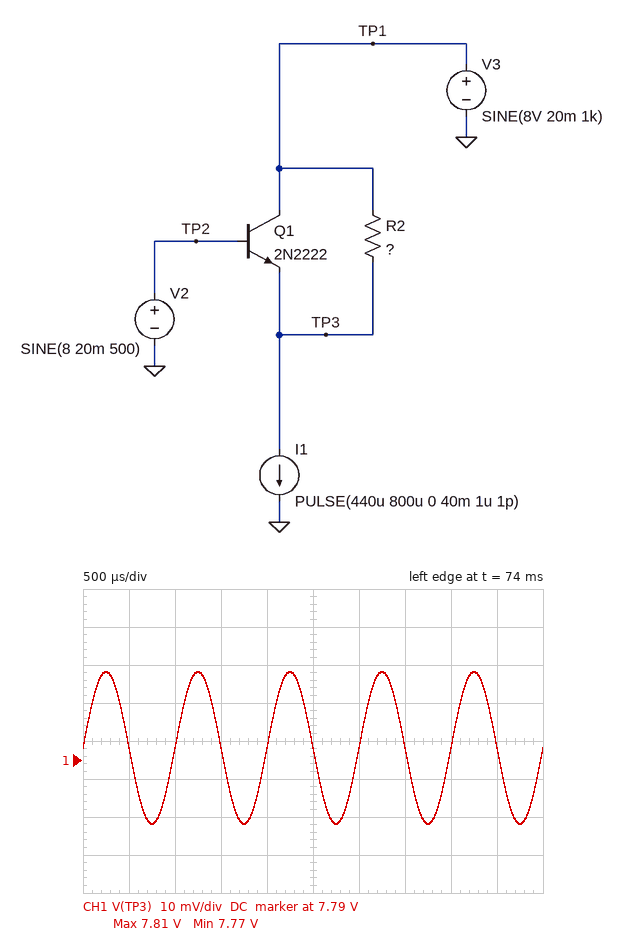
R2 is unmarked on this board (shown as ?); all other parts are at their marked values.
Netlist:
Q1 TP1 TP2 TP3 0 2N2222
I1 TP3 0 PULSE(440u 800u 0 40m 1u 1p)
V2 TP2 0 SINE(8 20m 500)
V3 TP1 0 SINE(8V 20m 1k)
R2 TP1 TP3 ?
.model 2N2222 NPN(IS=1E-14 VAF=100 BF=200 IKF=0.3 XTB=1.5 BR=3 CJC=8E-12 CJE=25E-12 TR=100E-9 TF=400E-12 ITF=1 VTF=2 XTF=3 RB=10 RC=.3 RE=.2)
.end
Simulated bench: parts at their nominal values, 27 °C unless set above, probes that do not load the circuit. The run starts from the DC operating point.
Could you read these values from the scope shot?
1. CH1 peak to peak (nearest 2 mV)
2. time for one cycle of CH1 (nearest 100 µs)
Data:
40 mV
1.0 ms
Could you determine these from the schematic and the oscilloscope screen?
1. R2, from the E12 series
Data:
470 Ω
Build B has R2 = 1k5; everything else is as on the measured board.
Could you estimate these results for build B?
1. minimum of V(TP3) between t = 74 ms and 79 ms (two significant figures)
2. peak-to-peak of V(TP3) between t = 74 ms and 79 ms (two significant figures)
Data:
7.4 V
35 mV
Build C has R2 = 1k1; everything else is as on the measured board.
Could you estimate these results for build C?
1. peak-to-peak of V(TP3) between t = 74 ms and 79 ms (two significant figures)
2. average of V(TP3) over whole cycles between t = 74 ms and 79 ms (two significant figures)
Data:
39 mV
7.5 V
